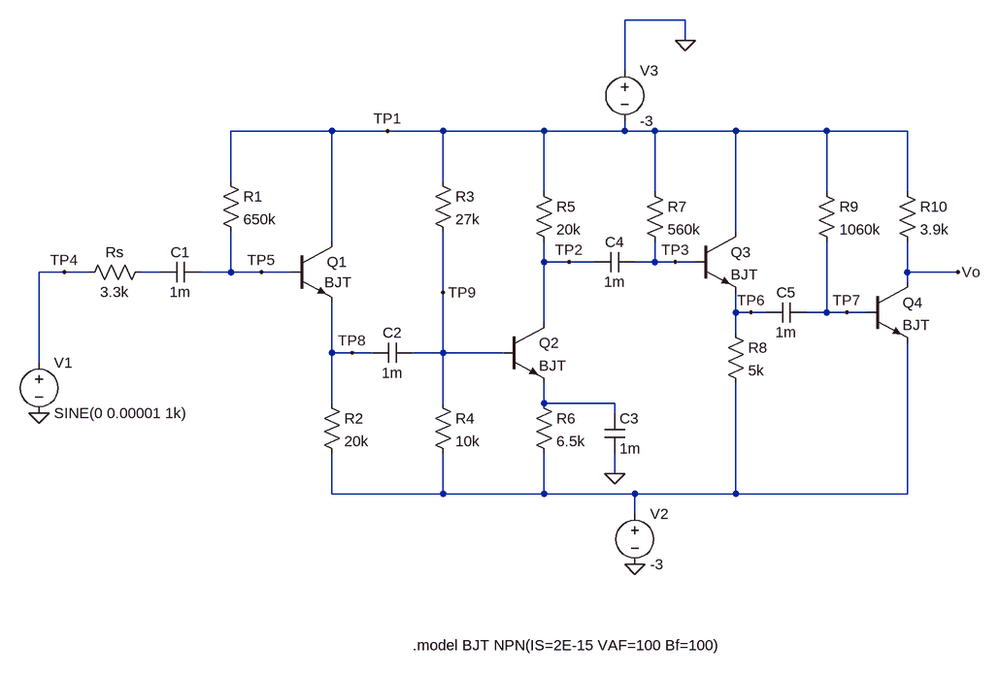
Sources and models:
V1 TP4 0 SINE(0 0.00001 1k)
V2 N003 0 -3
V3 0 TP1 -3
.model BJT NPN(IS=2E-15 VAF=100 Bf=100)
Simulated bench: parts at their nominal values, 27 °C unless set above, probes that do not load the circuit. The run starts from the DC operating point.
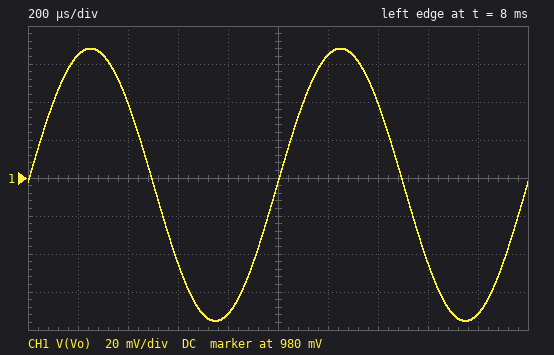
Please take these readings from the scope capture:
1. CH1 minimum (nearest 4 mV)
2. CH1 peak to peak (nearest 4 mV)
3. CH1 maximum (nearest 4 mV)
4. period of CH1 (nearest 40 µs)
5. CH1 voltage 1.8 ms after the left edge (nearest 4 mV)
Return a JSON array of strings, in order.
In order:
["904 mV", "144 mV", "1.048 V", "1.00 ms", "908 mV"]
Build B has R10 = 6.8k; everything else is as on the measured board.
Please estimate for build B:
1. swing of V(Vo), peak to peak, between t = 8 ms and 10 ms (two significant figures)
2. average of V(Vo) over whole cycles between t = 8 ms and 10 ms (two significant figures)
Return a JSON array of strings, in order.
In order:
["240 mV", "-480 mV"]
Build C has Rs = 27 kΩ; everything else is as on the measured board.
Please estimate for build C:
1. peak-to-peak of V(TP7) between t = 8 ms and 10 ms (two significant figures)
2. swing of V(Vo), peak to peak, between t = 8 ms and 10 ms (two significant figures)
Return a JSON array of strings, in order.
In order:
["1.7 mV", "130 mV"]
